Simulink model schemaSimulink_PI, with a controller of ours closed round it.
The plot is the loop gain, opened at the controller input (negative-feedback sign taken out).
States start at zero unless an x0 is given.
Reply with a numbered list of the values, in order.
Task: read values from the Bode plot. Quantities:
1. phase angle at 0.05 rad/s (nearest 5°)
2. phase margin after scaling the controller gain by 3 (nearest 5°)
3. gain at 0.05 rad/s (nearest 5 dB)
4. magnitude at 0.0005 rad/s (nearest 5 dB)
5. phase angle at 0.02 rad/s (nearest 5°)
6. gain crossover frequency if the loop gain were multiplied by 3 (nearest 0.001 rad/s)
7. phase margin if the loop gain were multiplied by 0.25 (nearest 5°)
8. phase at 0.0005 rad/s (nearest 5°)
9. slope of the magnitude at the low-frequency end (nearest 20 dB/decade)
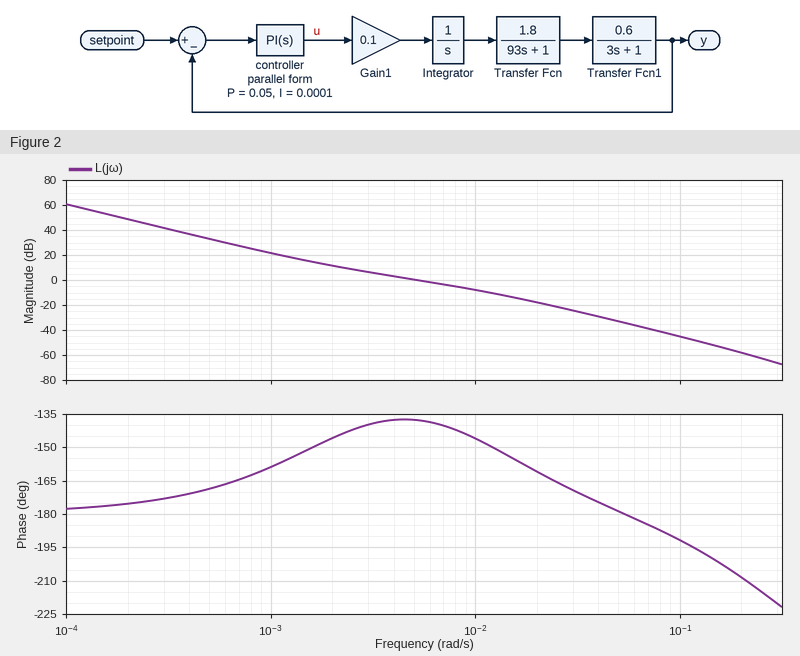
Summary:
1. -180°
2. 30°
3. -35 dB
4. 35 dB
5. -160°
6. 0.011 rad/s
7. 35°
8. -170°
9. -40 dB/decade
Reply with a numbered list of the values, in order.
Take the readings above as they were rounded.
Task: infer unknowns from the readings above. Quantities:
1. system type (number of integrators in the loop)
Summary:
1. 2
